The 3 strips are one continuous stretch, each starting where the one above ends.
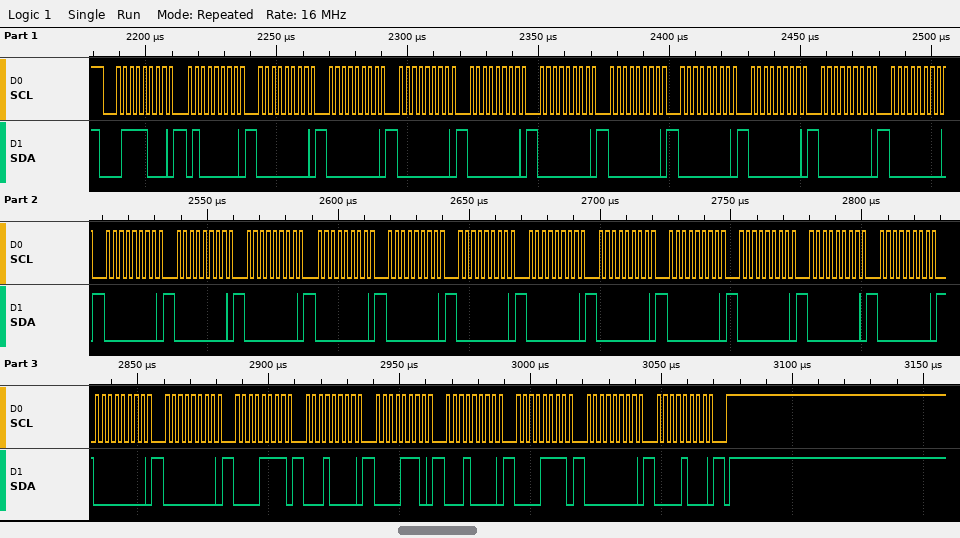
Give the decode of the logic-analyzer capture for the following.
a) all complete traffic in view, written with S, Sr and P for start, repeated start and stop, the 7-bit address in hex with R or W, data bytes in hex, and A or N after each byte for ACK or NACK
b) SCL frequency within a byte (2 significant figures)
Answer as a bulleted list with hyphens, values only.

- S 3CW A 40 A 00 A 00 A 00 A 00 A 00 A 00 A 00 A 00 A 00 A 00 A 00 A 00 A 00 A 00 A 00 A 00 A 00 A 00 A 00 A 00 A 00 A 00 A 00 A 00 A 0F A 10 A 0E A 10 A 0F A 00 A 08 A P
- 400 kHz
